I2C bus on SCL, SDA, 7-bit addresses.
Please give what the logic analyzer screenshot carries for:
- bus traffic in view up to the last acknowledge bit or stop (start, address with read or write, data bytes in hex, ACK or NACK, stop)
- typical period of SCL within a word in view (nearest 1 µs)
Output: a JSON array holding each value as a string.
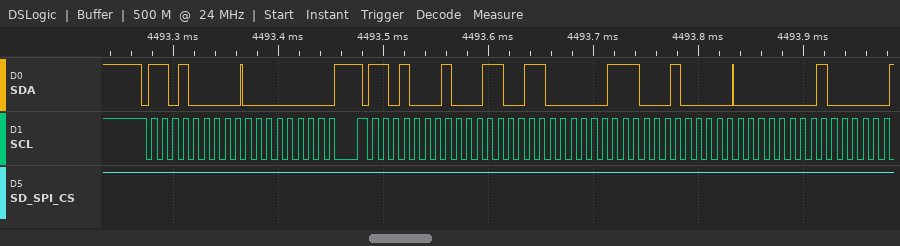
["start, address 68 write ACK, 00 ACK, repeated start, address 68 read ACK, 33 ACK, 07 ACK, 20 ACK, 01 ACK", "10 µs"]
